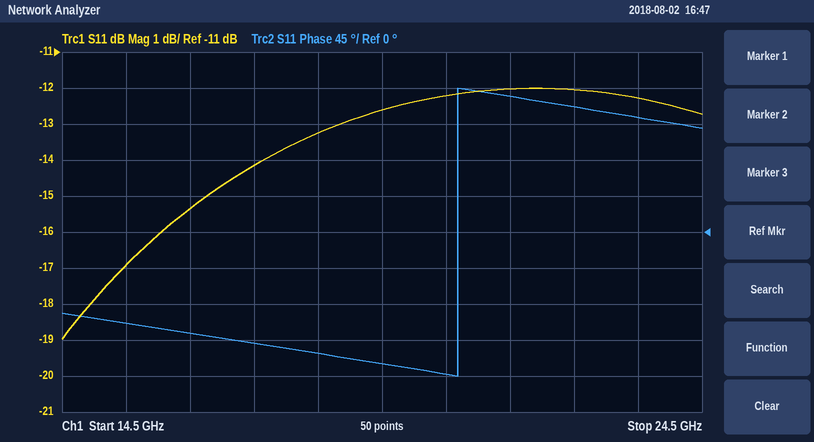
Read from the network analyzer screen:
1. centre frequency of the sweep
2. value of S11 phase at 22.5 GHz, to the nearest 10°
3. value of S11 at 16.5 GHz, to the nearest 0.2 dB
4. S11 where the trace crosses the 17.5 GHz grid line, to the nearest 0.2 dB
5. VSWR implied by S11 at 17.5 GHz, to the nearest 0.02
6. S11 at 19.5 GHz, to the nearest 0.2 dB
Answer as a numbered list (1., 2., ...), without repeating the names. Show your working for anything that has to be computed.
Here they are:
1. 19.5 GHz
2. 160°
3. -15.4 dB
4. -14.2 dB
5. |Γ| = 10^(-14.2/20) = 0.1950; VSWR = (1 + 0.1950)/(1 − 0.1950) ≈ 1.48
6. -12.6 dB
